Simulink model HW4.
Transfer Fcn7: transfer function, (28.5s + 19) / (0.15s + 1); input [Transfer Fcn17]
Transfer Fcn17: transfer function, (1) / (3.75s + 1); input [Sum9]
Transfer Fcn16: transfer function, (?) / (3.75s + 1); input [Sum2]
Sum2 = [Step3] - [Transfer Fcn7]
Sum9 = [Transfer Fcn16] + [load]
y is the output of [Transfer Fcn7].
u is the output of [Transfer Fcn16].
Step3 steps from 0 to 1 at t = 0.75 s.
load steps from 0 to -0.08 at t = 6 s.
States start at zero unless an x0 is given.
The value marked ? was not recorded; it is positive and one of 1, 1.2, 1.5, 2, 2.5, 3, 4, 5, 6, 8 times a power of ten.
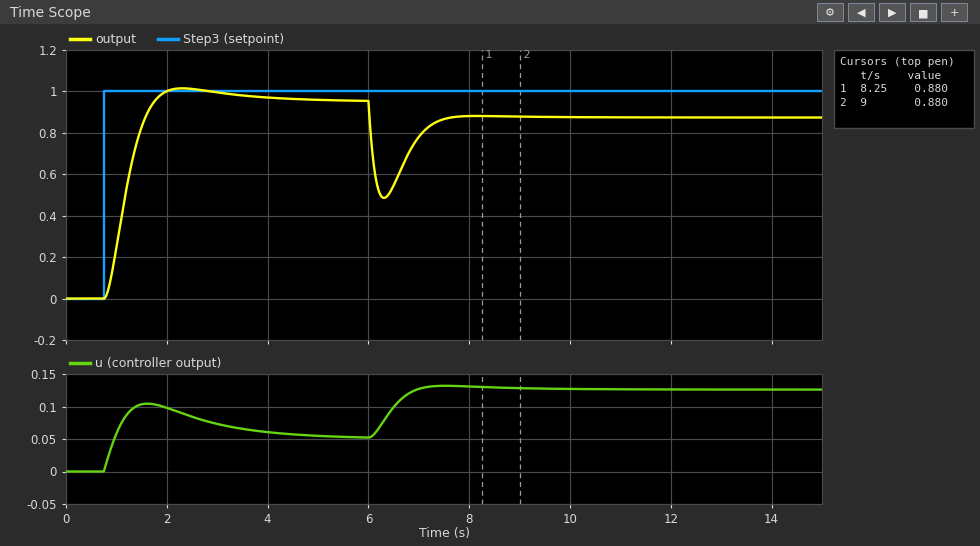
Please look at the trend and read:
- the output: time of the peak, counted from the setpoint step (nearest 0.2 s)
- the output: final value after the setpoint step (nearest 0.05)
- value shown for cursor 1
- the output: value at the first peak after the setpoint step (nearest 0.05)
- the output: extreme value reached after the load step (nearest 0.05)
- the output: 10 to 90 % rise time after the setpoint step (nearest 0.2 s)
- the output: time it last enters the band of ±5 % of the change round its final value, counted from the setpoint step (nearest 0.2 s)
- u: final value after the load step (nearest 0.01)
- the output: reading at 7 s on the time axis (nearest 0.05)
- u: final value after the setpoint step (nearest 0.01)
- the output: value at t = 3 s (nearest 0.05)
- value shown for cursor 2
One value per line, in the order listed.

1.6 s
0.95
0.880
1.00
0.50
0.6 s
2.2 s
0.13
0.80
0.05
1.00
0.880
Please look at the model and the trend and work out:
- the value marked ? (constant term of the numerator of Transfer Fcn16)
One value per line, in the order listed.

1
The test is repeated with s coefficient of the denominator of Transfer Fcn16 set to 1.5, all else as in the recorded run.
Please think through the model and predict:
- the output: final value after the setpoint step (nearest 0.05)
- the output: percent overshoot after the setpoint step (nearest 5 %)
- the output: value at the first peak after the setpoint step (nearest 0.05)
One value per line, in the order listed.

0.95
10 %
1.05
